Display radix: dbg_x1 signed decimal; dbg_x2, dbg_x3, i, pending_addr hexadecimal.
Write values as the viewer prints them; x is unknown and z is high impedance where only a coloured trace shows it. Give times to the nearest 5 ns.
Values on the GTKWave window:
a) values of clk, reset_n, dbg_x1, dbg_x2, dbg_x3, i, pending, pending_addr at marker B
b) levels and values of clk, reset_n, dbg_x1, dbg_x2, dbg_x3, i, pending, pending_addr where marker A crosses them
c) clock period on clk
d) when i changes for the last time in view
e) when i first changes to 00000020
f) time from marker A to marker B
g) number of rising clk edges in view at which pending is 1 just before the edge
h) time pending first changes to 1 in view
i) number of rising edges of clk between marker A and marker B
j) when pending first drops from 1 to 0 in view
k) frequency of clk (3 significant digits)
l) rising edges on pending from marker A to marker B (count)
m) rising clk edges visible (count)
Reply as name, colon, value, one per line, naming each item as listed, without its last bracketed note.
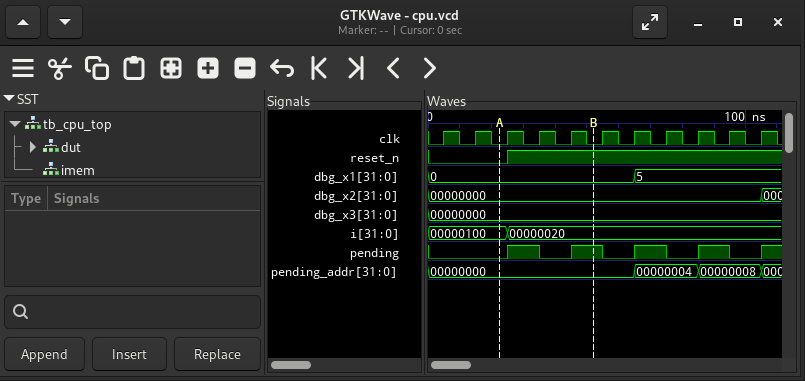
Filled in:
values of clk, reset_n, dbg_x1, dbg_x2, dbg_x3, i, pending, pending_addr at marker B: clk=0, reset_n=1, dbg_x1=0, dbg_x2=00000000, dbg_x3=00000000, i=00000020, pending=1, pending_addr=00000000
levels and values of clk, reset_n, dbg_x1, dbg_x2, dbg_x3, i, pending, pending_addr where marker A crosses them: clk=0, reset_n=0, dbg_x1=0, dbg_x2=00000000, dbg_x3=00000000, i=00000100, pending=0, pending_addr=00000000
clock period on clk: 10 ns
when i changes for the last time in view: 25 ns
when i first changes to 00000020: 25 ns
time from marker A to marker B: 30 ns
number of rising clk edges in view at which pending is 1 just before the edge: 4
time pending first changes to 1 in view: 25 ns
number of rising edges of clk between marker A and marker B: 3
when pending first drops from 1 to 0 in view: 35 ns
frequency of clk: 100 MHz
rising edges on pending from marker A to marker B: 2
rising clk edges visible: 11
